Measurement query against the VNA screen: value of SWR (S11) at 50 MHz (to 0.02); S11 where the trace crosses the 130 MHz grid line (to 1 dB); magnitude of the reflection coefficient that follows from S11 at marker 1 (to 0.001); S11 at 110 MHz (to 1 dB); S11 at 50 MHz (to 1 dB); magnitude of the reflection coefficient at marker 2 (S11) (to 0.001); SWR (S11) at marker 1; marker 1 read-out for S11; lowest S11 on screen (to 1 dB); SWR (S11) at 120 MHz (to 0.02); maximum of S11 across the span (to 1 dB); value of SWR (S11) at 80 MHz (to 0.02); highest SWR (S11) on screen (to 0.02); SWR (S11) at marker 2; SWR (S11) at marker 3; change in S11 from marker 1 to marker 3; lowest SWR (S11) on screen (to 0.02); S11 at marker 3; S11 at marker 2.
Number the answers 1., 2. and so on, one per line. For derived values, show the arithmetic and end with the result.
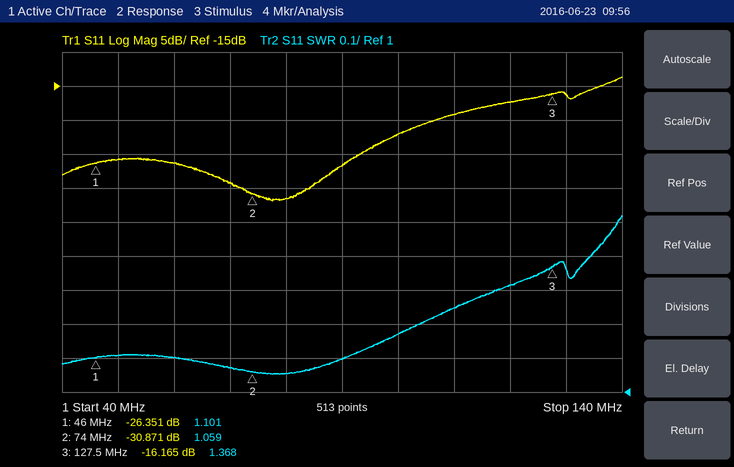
1. 1.10
2. -16 dB
3. 10^(-26.351/20) ≈ 0.048
4. -19 dB
5. -26 dB
6. 10^(-30.871/20) ≈ 0.029
7. 1.101
8. -26.351 dB
9. -32 dB
10. 1.32
11. -14 dB
12. 1.06
13. 1.52
14. 1.059
15. 1.368
16. -16.165 − (-26.351) = 10.186 dB
17. 1.06
18. -16.165 dB
19. -30.871 dB
